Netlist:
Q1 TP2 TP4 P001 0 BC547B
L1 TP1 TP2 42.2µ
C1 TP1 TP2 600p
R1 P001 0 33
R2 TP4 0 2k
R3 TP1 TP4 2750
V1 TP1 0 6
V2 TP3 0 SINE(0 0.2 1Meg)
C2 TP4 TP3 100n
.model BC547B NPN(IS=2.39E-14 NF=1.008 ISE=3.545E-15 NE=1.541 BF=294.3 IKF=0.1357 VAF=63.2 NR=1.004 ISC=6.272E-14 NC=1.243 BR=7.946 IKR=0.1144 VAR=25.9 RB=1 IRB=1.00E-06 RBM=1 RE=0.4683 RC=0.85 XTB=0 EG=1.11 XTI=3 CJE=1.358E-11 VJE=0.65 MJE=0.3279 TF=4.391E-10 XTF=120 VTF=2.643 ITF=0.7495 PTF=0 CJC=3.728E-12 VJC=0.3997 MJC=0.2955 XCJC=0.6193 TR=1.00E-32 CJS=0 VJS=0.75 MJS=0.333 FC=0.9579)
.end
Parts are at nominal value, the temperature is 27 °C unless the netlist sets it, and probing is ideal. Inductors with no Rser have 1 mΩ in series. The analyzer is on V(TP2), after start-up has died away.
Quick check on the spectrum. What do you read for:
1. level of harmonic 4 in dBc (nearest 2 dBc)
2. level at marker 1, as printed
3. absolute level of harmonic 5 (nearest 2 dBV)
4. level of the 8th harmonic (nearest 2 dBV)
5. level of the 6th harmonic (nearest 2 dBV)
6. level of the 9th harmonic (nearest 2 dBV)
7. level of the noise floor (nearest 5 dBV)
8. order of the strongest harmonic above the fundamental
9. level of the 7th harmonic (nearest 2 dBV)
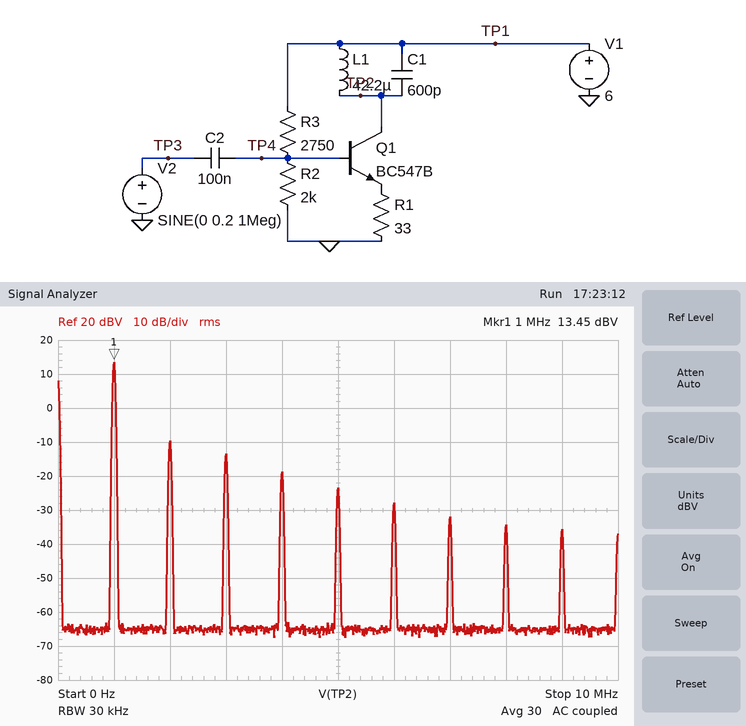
-32 dBc
13.45 dBV
-24 dBV
-34 dBV
-28 dBV
-36 dBV
-65 dBV
2
-32 dBV
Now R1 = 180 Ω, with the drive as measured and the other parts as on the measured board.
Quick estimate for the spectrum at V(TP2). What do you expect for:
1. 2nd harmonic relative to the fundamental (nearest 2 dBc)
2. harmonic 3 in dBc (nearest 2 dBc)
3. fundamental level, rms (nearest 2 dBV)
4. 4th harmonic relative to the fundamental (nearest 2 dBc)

-28 dBc
-34 dBc
10 dBV
-38 dBc
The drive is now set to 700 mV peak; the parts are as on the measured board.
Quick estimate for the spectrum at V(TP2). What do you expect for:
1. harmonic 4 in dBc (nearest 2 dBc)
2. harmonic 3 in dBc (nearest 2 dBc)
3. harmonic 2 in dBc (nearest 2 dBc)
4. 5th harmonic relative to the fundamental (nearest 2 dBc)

-30 dBc
-30 dBc
-30 dBc
-34 dBc
